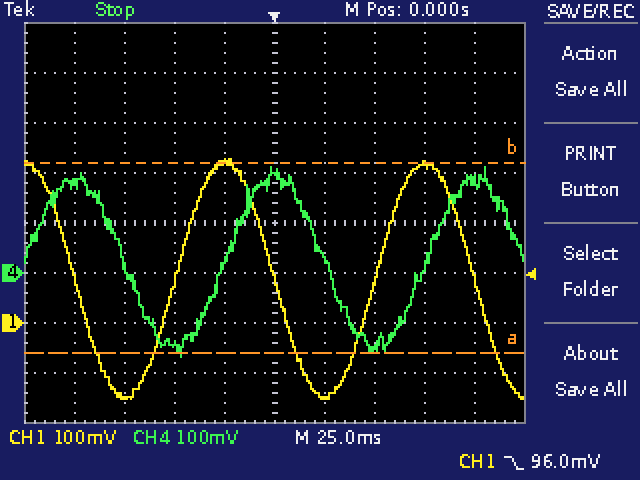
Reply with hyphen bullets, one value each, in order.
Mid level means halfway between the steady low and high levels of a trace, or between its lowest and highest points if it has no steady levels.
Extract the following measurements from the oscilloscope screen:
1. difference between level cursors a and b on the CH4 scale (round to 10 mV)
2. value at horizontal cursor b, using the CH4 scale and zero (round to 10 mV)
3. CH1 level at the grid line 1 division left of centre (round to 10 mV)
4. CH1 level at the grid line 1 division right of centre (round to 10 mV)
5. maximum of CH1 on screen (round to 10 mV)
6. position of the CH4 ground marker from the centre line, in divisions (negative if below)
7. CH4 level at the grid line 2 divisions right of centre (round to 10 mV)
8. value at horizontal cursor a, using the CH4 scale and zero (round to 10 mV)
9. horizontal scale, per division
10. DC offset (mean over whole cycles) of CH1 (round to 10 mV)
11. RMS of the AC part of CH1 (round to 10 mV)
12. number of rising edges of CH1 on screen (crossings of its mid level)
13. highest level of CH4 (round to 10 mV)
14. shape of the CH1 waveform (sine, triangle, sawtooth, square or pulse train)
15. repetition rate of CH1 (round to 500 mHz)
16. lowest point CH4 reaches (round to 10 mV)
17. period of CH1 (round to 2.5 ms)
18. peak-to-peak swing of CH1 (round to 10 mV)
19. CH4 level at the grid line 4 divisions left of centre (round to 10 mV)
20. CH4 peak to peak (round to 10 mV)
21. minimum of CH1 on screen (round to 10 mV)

- 380 mV
- 220 mV
- 320 mV
- -150 mV
- 330 mV
- -1.0 div
- -150 mV
- -160 mV
- 25 ms
- 90 mV
- 170 mV
- 2
- 210 mV
- sine
- 10.0 Hz
- -170 mV
- 100.0 ms
- 480 mV
- 180 mV
- 380 mV
- -150 mV
